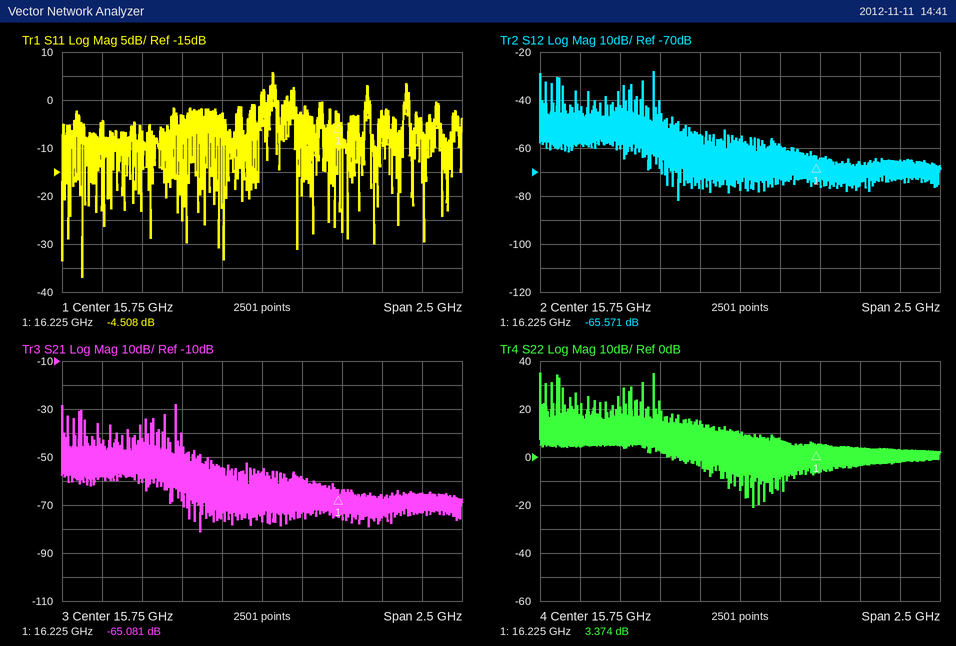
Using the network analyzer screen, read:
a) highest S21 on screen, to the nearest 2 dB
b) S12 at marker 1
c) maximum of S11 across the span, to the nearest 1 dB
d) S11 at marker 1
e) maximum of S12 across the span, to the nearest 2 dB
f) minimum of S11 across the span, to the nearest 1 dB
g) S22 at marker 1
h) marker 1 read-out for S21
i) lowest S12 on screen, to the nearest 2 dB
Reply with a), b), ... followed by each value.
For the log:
a) -28 dB
b) -65.571 dB
c) 6 dB
d) -4.508 dB
e) -28 dB
f) -37 dB
g) 3.374 dB
h) -65.081 dB
i) -82 dB
